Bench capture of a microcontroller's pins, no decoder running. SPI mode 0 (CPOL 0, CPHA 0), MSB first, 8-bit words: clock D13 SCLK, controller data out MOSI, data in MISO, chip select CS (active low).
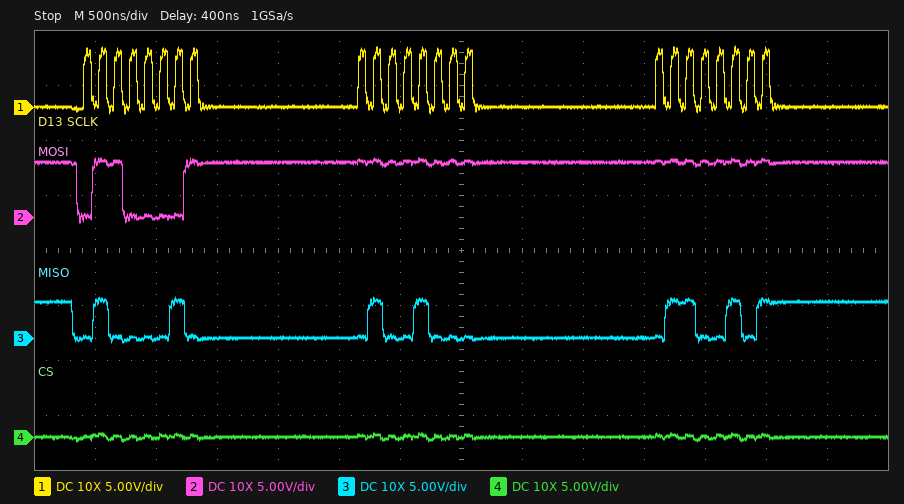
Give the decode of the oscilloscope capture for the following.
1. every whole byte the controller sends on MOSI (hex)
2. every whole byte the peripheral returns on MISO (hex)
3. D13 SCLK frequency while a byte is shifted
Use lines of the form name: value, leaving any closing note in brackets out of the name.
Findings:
every whole byte the controller sends on MOSI: 0x61 0xFF 0xFF
every whole byte the peripheral returns on MISO: 0x42 0x48 0x65
D13 SCLK frequency while a byte is shifted: 8 MHz
